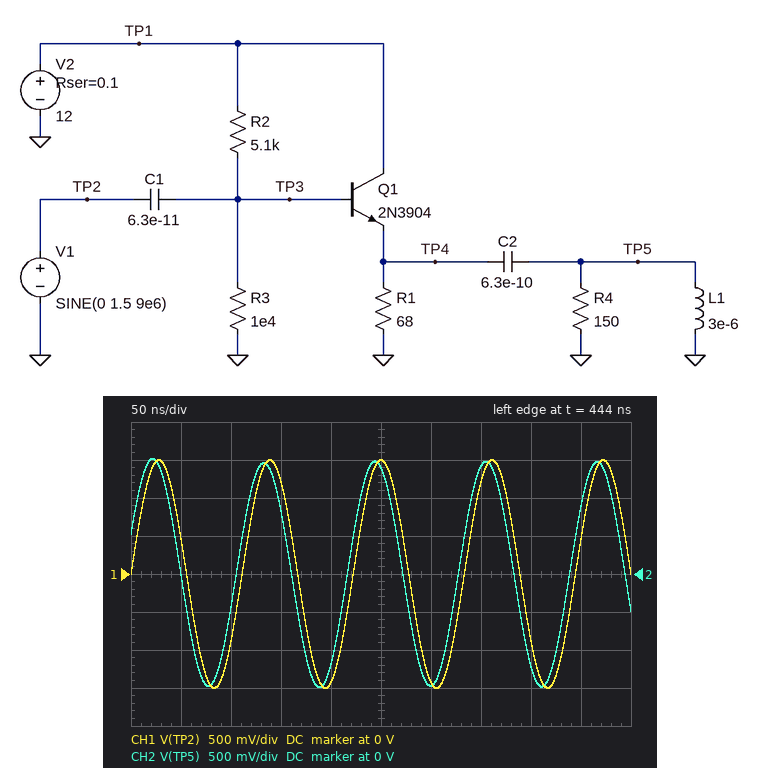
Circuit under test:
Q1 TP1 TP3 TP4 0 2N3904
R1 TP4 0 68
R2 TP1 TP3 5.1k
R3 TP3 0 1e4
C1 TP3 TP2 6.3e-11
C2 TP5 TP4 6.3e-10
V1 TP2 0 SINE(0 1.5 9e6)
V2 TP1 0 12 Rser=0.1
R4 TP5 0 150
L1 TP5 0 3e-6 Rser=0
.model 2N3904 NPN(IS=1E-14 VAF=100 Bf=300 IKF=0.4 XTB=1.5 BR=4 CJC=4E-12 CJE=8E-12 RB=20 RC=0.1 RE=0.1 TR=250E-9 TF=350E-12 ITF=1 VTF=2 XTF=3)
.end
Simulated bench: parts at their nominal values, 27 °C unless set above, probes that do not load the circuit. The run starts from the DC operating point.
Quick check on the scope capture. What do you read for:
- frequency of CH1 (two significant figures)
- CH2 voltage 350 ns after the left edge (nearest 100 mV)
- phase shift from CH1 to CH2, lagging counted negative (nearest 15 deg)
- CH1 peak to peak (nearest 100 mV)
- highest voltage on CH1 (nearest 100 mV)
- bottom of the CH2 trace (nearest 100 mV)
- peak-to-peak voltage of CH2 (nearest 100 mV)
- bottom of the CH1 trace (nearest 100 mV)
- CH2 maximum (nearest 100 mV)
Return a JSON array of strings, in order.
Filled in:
["9.0 MHz", "1.4 V", "15 deg", "3.0 V", "1.5 V", "-1.5 V", "3.0 V", "-1.5 V", "1.5 V"]
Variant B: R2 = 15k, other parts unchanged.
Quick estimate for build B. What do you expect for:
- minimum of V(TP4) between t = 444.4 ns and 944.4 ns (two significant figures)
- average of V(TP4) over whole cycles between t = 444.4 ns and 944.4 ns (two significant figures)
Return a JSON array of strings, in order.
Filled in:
["1.8 V", "3.1 V"]
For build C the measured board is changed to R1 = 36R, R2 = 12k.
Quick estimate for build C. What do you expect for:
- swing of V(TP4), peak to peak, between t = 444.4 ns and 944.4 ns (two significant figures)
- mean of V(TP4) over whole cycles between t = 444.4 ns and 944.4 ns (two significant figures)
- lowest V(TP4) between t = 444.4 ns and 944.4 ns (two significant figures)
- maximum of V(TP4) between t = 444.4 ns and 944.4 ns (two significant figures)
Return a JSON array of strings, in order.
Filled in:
["2.4 V", "3.0 V", "1.8 V", "4.2 V"]
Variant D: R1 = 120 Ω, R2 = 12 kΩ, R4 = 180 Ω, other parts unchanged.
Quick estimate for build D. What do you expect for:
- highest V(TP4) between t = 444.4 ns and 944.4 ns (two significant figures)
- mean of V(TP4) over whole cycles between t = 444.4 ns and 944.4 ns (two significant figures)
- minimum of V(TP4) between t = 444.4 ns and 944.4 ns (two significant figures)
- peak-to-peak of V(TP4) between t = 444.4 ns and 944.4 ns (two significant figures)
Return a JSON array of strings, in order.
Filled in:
["5.4 V", "4.1 V", "2.7 V", "2.6 V"]
